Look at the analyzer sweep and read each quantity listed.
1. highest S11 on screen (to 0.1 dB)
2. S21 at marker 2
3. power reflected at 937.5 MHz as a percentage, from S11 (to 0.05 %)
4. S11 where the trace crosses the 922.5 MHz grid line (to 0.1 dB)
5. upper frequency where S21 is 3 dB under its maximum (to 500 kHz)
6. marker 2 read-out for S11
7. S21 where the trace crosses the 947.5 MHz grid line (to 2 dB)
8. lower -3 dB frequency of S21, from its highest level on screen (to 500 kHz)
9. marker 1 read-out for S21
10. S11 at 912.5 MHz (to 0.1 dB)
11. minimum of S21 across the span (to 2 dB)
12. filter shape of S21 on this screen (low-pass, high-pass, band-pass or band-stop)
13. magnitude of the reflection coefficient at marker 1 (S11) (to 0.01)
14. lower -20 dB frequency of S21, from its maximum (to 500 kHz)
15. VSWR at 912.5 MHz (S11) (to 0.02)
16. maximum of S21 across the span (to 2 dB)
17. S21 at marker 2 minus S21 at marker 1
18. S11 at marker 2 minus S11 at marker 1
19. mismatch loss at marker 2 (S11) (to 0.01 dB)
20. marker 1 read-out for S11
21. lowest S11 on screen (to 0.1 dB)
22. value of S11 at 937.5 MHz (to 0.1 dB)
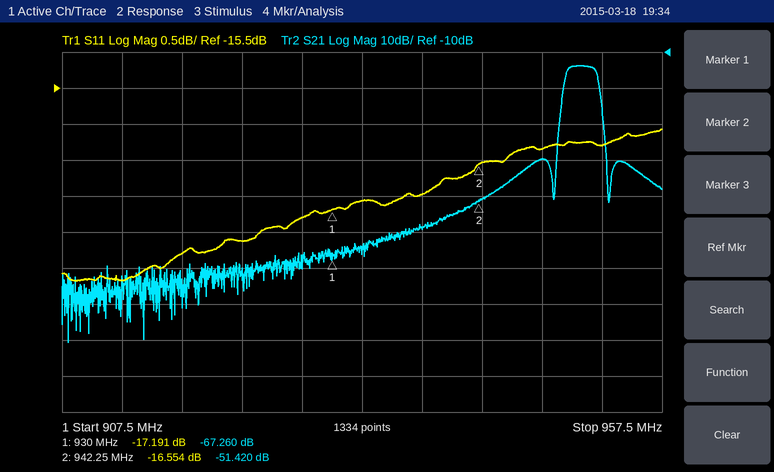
-16.1 dB
-51.420 dB
2.00 %
-17.6 dB
952.0 MHz
-16.554 dB
-40 dB
949.5 MHz
-67.260 dB
-18.2 dB
-90 dB
band-pass
0.14
949.0 MHz
1.28
-14 dB
15.840 dB
0.637 dB
0.10 dB
-17.191 dB
-18.2 dB
-17.0 dB
